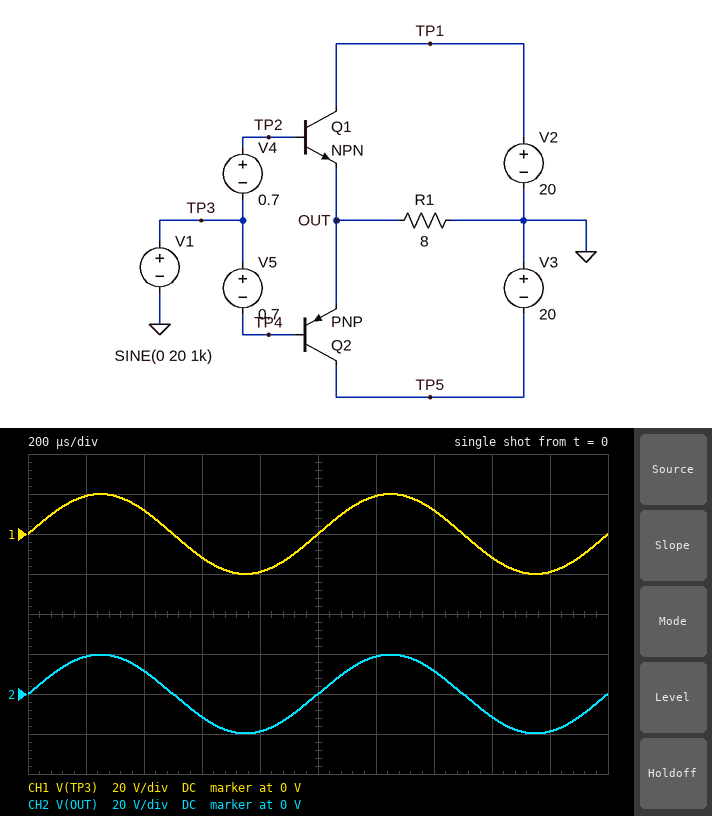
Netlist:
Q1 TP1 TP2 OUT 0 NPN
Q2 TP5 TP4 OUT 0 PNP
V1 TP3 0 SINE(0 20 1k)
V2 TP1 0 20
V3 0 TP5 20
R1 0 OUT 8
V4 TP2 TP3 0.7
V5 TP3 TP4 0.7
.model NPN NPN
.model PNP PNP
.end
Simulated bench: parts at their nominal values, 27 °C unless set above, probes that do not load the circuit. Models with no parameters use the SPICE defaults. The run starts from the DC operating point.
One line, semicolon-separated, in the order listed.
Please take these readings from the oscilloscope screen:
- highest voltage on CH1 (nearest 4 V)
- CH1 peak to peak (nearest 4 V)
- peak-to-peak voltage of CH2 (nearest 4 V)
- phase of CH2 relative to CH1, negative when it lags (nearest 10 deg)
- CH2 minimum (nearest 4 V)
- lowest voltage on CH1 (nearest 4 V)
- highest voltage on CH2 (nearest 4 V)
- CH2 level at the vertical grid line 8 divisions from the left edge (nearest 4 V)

20 V; 40 V; 40 V; 0 deg; -20 V; -20 V; 20 V; -12 V
